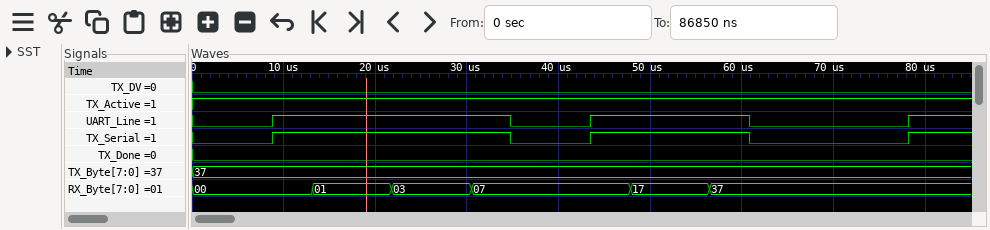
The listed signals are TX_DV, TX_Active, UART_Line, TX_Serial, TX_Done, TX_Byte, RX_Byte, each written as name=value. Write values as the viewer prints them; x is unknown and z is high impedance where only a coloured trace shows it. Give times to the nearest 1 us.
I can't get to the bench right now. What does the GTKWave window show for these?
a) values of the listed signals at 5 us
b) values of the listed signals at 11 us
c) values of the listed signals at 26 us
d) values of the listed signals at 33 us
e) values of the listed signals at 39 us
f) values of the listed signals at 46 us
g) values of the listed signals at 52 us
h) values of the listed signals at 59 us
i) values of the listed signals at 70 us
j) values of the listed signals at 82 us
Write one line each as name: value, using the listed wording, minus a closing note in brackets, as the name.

values of the listed signals at 5 us: TX_DV=0, TX_Active=1, UART_Line=0, TX_Serial=0, TX_Done=0, TX_Byte=37, RX_Byte=00
values of the listed signals at 11 us: TX_DV=0, TX_Active=1, UART_Line=1, TX_Serial=1, TX_Done=0, TX_Byte=37, RX_Byte=00
values of the listed signals at 26 us: TX_DV=0, TX_Active=1, UART_Line=1, TX_Serial=1, TX_Done=0, TX_Byte=37, RX_Byte=03
values of the listed signals at 33 us: TX_DV=0, TX_Active=1, UART_Line=1, TX_Serial=1, TX_Done=0, TX_Byte=37, RX_Byte=07
values of the listed signals at 39 us: TX_DV=0, TX_Active=1, UART_Line=0, TX_Serial=0, TX_Done=0, TX_Byte=37, RX_Byte=07
values of the listed signals at 46 us: TX_DV=0, TX_Active=1, UART_Line=1, TX_Serial=1, TX_Done=0, TX_Byte=37, RX_Byte=07
values of the listed signals at 52 us: TX_DV=0, TX_Active=1, UART_Line=1, TX_Serial=1, TX_Done=0, TX_Byte=37, RX_Byte=17
values of the listed signals at 59 us: TX_DV=0, TX_Active=1, UART_Line=1, TX_Serial=1, TX_Done=0, TX_Byte=37, RX_Byte=37
values of the listed signals at 70 us: TX_DV=0, TX_Active=1, UART_Line=0, TX_Serial=0, TX_Done=0, TX_Byte=37, RX_Byte=37
values of the listed signals at 82 us: TX_DV=0, TX_Active=1, UART_Line=1, TX_Serial=1, TX_Done=0, TX_Byte=37, RX_Byte=37
